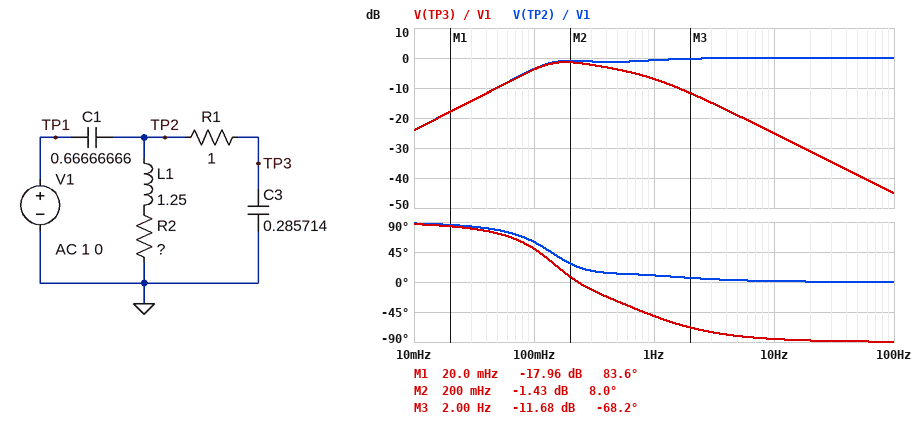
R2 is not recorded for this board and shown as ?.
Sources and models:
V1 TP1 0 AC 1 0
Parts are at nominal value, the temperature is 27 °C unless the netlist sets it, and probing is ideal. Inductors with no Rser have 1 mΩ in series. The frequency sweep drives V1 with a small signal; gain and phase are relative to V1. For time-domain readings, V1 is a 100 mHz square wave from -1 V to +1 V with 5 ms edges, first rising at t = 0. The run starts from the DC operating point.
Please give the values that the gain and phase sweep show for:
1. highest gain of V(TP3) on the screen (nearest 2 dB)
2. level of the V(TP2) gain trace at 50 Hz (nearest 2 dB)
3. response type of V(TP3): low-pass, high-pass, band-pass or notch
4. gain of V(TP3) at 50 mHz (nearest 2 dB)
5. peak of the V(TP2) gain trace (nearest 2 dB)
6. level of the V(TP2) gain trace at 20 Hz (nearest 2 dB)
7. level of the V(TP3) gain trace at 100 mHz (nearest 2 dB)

-2 dB
0 dB
band-pass
-10 dB
0 dB
0 dB
-4 dB
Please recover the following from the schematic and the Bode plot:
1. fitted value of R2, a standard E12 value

1.5 Ω
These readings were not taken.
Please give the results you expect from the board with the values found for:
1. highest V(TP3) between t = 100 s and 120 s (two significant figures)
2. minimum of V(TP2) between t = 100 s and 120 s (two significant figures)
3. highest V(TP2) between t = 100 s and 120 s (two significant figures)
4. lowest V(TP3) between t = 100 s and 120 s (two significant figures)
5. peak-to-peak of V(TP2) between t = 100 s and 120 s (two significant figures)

1.3 V
-2.1 V
2.1 V
-1.3 V
4.1 V
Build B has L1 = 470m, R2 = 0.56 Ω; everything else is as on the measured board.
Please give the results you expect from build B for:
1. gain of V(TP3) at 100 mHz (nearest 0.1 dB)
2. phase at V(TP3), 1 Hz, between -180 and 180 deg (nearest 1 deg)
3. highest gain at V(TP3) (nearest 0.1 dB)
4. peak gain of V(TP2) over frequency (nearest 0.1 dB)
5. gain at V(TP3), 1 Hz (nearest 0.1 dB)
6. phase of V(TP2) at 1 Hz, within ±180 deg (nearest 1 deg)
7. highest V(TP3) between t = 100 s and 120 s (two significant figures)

-10.8 dB
-50 deg
-0.2 dB
0.9 dB
-6.6 dB
11 deg
1.1 V
